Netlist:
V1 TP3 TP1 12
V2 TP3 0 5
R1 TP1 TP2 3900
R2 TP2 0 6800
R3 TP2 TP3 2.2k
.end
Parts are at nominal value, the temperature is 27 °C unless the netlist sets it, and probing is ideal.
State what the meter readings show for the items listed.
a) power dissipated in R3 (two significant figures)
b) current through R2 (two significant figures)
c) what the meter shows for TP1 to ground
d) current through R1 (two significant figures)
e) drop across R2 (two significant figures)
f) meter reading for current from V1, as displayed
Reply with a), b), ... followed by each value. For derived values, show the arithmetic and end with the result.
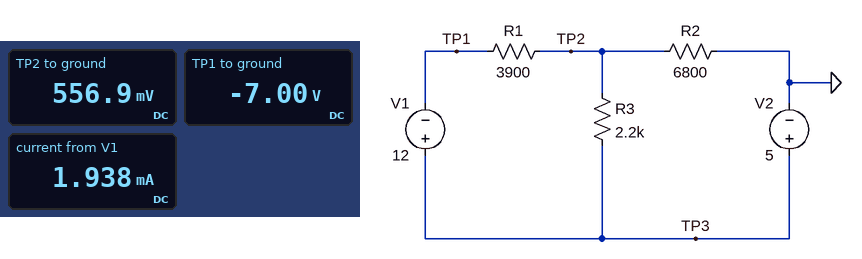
a) (5 V - 556.9 mV)^2 / 2.2 kΩ = 9.0 mW
b) (556.9 mV) / 6.8 kΩ = 82 µA
c) -7.00 V
d) (556.9 mV - (-7 V)) / 3.9 kΩ = 1.9 mA
e) 556.9 mV = 560 mV
f) 1.938 mA
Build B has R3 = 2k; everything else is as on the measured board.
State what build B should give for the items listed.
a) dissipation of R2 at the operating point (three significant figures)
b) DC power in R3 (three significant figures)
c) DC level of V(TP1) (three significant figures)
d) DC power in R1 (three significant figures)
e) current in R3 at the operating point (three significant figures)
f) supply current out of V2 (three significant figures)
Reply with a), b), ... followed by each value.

a) 89.6 µW
b) 8.90 mW
c) -7.00 V
d) 15.5 mW
e) 2.11 mA
f) 115 µA
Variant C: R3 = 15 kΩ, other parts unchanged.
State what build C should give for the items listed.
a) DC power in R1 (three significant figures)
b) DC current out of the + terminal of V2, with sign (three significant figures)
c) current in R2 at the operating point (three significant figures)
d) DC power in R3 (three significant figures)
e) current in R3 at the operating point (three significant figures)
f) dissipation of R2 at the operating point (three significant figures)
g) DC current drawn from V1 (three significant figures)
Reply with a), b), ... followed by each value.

a) 3.88 mW
b) -457 µA
c) 457 µA
d) 4.38 mW
e) 541 µA
f) 1.42 mW
g) 998 µA
